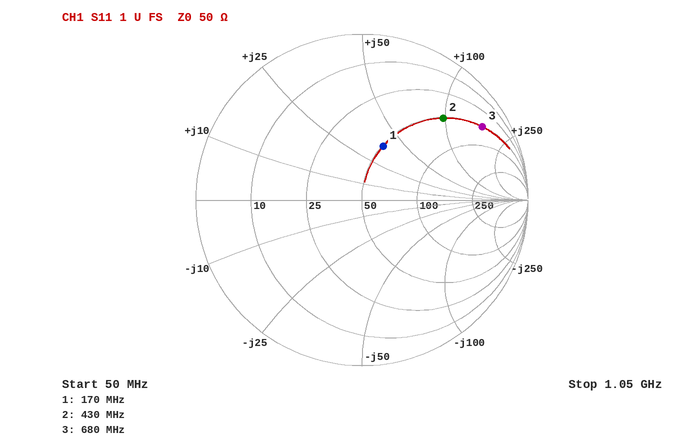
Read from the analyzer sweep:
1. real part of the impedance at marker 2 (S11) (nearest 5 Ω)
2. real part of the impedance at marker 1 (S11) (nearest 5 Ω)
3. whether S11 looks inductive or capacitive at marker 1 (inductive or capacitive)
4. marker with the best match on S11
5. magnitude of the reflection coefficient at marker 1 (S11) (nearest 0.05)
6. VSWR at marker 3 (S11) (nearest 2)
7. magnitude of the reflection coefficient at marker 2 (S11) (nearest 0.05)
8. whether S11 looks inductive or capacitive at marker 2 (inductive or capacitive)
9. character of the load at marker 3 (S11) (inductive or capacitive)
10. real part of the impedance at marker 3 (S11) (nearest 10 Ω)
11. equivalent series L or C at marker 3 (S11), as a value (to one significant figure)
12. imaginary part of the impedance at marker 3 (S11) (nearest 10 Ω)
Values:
50 Ω
50 Ω
inductive
marker 1
0.35
12
0.70
inductive
inductive
50 Ω
40 nH
+160 Ω
